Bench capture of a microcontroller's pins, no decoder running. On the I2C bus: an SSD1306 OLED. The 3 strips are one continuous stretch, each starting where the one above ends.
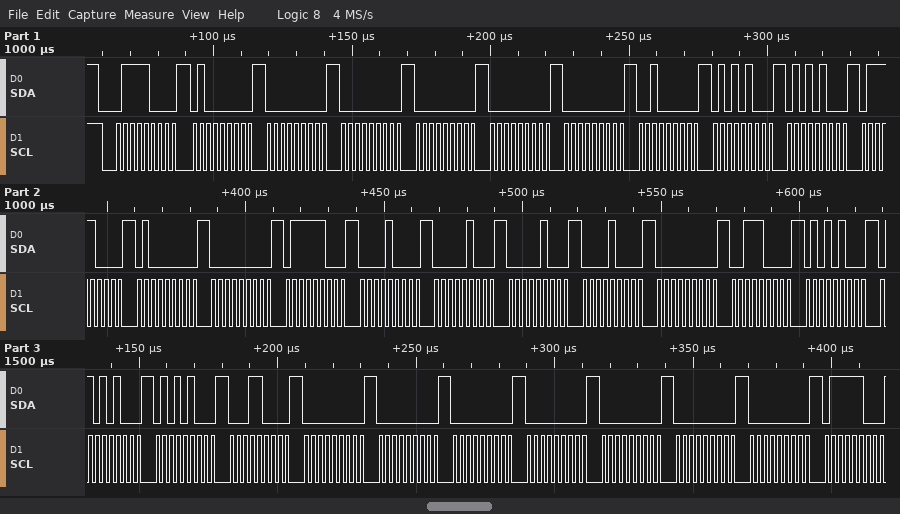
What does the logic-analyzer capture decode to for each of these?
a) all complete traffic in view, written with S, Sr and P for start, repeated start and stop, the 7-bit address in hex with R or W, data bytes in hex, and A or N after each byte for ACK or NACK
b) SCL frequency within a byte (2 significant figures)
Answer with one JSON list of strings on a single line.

["S 3CW A 40 A 00 A 00 A 00 A 00 A 00 A 20 A 54 A 54 A 78 A 40 A 00 A 7C A 08 A 04 A 04 A 08 A 00 A 38 A 54 A 54 A 54 A 18 A 00 A 00 A 00 A 00 A 00 A 00 A 00 A 7C A", "400 kHz"]
